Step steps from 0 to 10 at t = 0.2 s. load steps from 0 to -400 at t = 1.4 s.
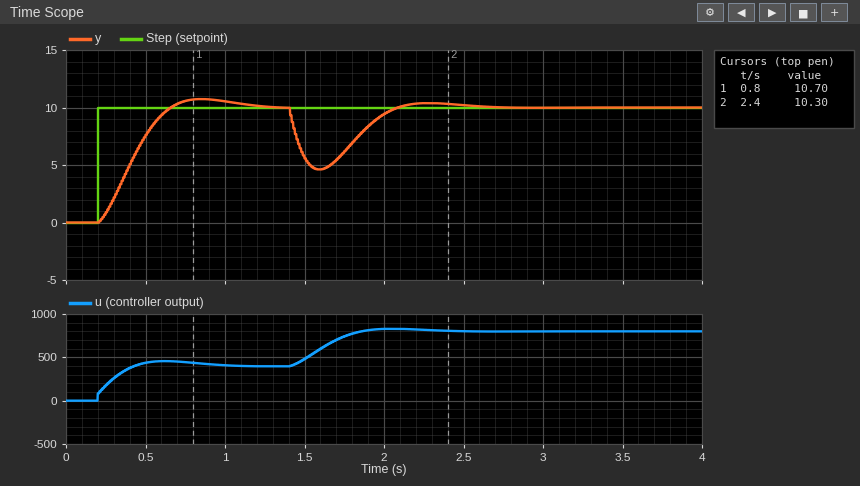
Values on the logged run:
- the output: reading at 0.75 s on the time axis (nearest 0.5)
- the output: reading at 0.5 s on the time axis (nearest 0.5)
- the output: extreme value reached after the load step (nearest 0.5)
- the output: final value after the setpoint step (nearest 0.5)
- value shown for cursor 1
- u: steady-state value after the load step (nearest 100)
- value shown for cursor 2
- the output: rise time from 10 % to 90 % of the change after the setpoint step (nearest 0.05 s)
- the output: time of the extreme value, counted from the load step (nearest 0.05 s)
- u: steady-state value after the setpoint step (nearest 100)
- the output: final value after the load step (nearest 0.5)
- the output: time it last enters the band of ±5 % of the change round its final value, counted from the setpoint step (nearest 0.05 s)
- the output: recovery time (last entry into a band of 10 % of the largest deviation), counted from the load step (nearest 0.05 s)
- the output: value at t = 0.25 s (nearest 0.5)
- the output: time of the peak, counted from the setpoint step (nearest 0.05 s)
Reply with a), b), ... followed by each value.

a) 10.5
b) 7.5
c) 4.5
d) 10.0
e) 10.70
f) 800
g) 10.30
h) 0.30 s
i) 0.20 s
j) 400
k) 10.0
l) 0.80 s
m) 0.60 s
n) 1.0
o) 0.65 s
